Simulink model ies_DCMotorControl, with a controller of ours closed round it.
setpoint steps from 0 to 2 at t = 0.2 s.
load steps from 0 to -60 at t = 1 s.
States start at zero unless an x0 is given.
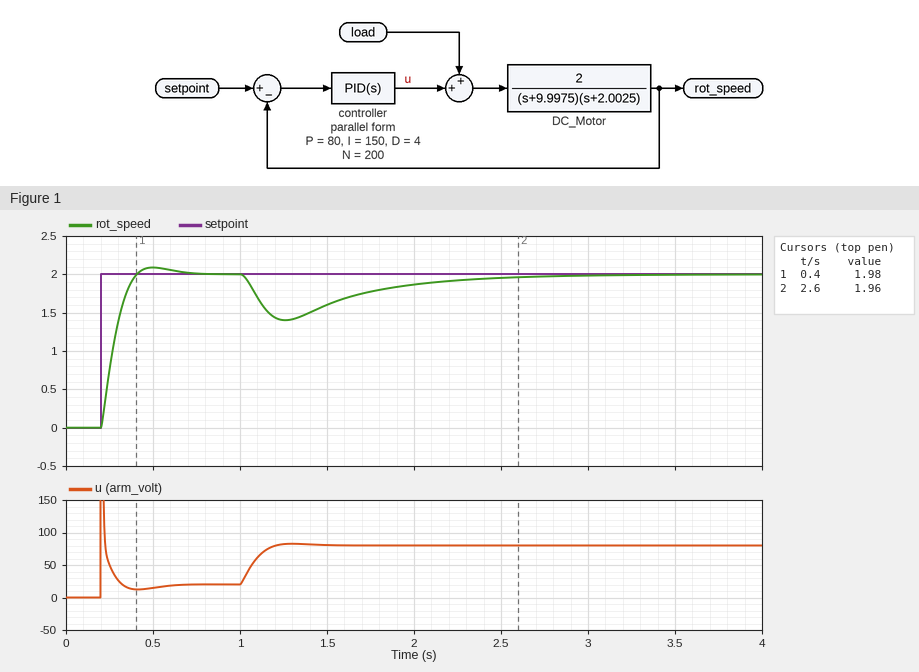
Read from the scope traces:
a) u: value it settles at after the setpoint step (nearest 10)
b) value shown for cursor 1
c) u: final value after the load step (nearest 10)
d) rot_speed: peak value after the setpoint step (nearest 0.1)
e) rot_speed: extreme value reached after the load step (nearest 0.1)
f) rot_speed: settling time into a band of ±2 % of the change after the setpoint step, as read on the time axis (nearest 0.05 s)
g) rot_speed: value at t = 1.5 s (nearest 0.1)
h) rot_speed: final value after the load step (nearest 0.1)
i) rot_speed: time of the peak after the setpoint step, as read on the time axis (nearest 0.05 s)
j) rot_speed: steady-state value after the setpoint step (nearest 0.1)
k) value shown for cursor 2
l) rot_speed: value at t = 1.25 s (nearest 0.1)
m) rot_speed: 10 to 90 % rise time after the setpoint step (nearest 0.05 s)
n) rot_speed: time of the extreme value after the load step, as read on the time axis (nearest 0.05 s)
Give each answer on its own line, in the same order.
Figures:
20
1.98
80
2.1
1.4
0.65 s
1.6
2.0
0.50 s
2.0
1.96
1.4
0.15 s
1.25 s
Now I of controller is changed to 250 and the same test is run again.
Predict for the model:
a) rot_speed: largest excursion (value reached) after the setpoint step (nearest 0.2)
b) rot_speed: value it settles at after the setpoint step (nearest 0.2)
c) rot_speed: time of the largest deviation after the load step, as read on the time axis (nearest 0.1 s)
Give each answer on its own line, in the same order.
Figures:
2.2
2.0
1.2 s
